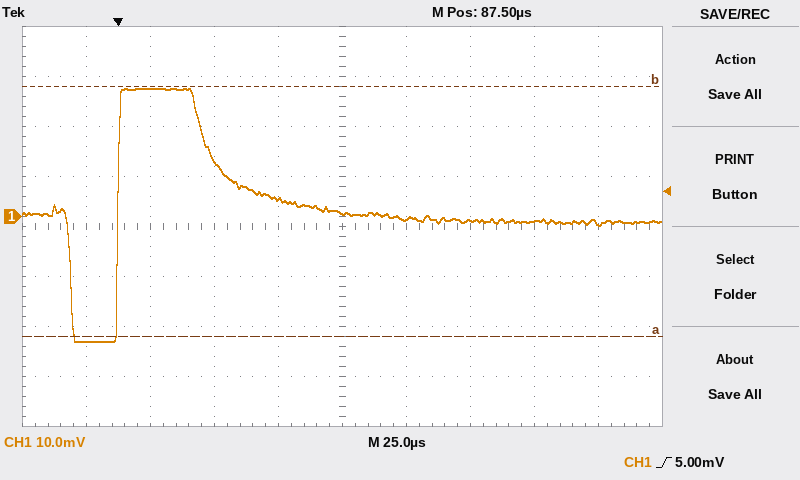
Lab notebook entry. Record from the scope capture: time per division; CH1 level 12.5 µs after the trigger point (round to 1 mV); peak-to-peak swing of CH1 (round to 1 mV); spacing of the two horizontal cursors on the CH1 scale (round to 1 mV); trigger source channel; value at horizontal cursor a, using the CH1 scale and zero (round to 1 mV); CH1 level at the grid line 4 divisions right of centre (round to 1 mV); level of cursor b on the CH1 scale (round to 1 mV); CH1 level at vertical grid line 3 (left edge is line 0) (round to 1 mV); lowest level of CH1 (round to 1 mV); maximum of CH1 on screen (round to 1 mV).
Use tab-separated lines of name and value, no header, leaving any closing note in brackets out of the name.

time per division	25 µs
CH1 level 12.5 µs after the trigger point	26 mV
peak-to-peak swing of CH1	51 mV
spacing of the two horizontal cursors on the CH1 scale	50 mV
trigger source channel	CH1
value at horizontal cursor a, using the CH1 scale and zero	-24 mV
CH1 level at the grid line 4 divisions right of centre	-1 mV
level of cursor b on the CH1 scale	26 mV
CH1 level at vertical grid line 3 (left edge is line 0)	11 mV
lowest level of CH1	-25 mV
maximum of CH1 on screen	26 mV
